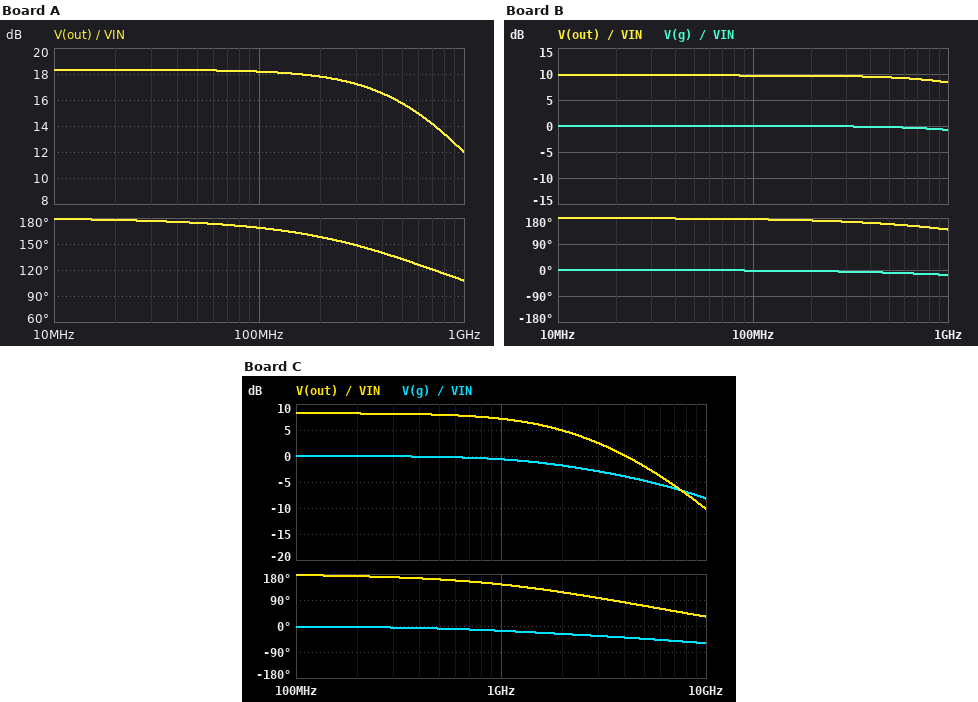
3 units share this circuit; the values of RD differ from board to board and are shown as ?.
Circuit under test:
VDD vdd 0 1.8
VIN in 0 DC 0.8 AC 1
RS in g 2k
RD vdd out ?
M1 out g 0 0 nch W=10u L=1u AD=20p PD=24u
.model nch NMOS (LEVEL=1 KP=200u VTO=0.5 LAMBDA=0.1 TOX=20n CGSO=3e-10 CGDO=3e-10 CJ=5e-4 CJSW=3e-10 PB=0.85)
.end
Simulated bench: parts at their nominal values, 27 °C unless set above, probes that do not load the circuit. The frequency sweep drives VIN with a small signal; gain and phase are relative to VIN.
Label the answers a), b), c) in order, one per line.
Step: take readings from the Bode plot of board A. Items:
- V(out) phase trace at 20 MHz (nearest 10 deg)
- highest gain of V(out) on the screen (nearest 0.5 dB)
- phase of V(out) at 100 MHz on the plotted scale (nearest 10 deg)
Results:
a) 180 deg
b) 18.5 dB
c) 170 deg
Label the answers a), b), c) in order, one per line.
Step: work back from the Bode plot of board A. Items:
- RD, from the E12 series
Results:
a) 15 kΩ
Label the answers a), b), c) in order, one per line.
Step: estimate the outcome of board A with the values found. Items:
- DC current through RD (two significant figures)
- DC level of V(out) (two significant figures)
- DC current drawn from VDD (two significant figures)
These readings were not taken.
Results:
a) 94 µA
b) 400 mV
c) 94 µA
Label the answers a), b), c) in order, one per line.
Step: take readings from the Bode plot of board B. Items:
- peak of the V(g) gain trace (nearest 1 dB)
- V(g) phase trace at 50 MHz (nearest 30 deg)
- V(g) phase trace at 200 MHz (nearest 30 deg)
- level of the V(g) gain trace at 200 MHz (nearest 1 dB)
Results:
a) 0 dB
b) 0 deg
c) 0 deg
d) 0 dB
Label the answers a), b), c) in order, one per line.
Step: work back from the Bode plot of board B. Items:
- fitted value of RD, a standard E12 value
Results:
a) 4.7 kΩ
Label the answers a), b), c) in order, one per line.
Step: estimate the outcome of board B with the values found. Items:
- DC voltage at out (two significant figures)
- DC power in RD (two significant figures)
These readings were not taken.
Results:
a) 1.3 V
b) 49 µW
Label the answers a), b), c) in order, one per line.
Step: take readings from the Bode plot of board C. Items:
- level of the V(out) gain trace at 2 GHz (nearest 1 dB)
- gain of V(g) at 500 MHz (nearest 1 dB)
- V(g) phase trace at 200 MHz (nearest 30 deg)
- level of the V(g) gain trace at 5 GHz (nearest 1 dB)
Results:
a) 5 dB
b) 0 dB
c) 0 deg
d) -5 dB
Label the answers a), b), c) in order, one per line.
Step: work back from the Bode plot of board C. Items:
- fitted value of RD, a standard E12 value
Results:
a) 3.9 kΩ
